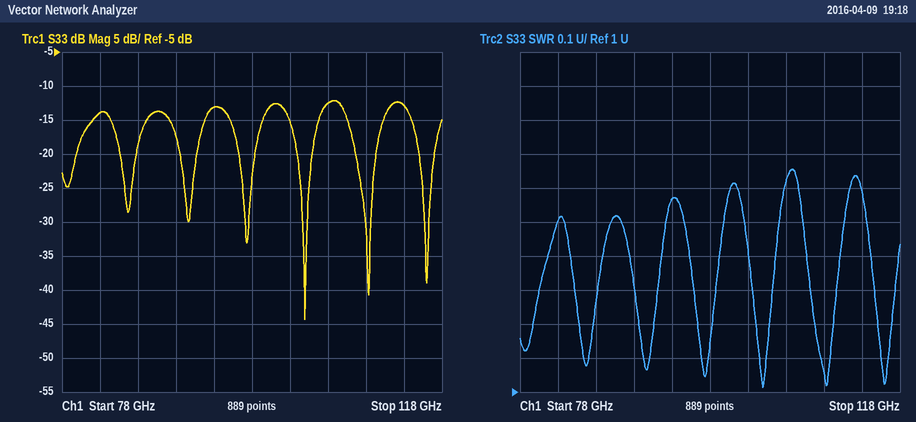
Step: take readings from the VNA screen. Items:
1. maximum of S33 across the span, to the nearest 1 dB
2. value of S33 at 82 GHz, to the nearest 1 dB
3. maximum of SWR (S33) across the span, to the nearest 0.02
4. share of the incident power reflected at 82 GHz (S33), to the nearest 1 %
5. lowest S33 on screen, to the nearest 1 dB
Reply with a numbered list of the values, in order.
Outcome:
1. -12 dB
2. -14 dB
3. 1.66
4. 4 %
5. -44 dB
